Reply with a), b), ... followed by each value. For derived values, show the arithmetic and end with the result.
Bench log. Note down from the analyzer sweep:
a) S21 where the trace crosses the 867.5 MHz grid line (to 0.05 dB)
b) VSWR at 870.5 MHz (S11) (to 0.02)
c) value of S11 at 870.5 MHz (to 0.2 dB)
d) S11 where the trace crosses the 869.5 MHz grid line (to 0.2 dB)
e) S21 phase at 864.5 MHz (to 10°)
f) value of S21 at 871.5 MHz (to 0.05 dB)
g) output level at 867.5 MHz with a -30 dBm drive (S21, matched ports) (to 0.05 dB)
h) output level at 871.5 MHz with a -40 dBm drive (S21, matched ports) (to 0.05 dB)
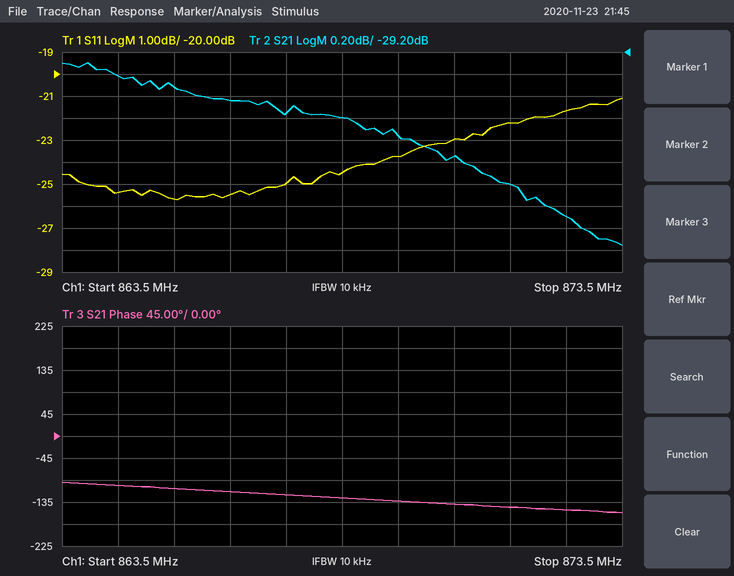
a) -29.75 dB
b) |Γ| = 10^(-23/20) = 0.0708; VSWR = (1 + 0.0708)/(1 − 0.0708) ≈ 1.15, so 1.16 to the nearest 0.02
c) -23.0 dB
d) -23.8 dB
e) -100°
f) -30.40 dB
g) -30 dBm + (-29.75 dB) = -59.75 dBm
h) -40 dBm + (-30.40 dB) = -70.40 dBm
